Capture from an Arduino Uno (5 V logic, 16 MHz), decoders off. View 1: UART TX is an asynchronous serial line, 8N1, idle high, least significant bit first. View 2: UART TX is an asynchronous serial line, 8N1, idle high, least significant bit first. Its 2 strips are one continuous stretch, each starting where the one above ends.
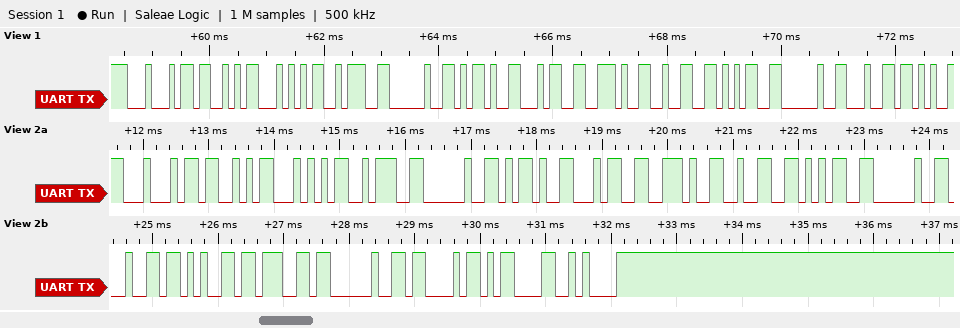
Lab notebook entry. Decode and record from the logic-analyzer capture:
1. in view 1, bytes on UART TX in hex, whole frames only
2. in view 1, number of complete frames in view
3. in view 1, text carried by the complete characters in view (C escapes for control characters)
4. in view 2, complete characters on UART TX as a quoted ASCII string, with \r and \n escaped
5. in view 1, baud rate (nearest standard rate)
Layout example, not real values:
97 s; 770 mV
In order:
44 53 54 3A 20 2D 34 2E 32 35 20 64; 12; "DST: -4.25 d"; "DST: -4.25 deg C\r\n"; 9600 baud
